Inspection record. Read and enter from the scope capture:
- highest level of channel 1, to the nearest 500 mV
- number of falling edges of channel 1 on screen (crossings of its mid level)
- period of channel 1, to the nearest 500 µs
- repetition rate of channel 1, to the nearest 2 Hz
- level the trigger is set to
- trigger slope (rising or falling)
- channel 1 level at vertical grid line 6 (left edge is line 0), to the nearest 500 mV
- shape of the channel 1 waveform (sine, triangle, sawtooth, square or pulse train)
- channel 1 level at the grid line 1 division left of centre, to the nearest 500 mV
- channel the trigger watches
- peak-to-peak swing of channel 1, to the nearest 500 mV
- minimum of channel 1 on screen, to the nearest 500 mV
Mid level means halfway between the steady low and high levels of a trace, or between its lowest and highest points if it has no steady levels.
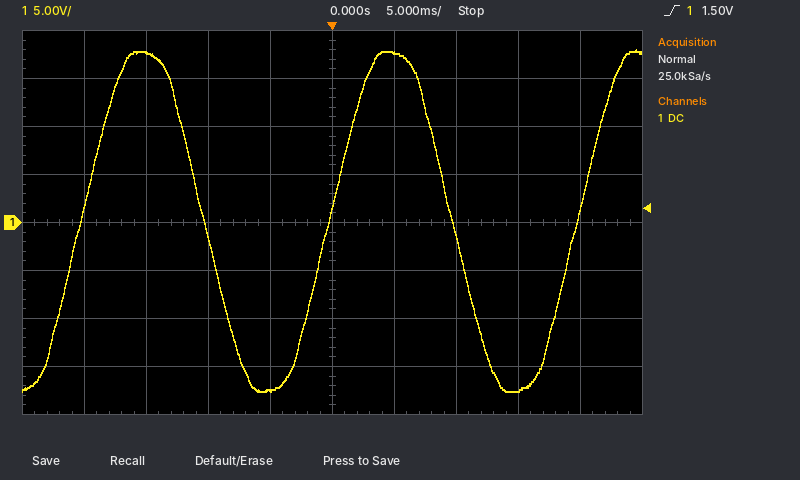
18.0 V
2
20.0 ms
50 Hz
1.50 V
rising
17.5 V
sine
-17.5 V
channel 1
35.5 V
-17.5 V
